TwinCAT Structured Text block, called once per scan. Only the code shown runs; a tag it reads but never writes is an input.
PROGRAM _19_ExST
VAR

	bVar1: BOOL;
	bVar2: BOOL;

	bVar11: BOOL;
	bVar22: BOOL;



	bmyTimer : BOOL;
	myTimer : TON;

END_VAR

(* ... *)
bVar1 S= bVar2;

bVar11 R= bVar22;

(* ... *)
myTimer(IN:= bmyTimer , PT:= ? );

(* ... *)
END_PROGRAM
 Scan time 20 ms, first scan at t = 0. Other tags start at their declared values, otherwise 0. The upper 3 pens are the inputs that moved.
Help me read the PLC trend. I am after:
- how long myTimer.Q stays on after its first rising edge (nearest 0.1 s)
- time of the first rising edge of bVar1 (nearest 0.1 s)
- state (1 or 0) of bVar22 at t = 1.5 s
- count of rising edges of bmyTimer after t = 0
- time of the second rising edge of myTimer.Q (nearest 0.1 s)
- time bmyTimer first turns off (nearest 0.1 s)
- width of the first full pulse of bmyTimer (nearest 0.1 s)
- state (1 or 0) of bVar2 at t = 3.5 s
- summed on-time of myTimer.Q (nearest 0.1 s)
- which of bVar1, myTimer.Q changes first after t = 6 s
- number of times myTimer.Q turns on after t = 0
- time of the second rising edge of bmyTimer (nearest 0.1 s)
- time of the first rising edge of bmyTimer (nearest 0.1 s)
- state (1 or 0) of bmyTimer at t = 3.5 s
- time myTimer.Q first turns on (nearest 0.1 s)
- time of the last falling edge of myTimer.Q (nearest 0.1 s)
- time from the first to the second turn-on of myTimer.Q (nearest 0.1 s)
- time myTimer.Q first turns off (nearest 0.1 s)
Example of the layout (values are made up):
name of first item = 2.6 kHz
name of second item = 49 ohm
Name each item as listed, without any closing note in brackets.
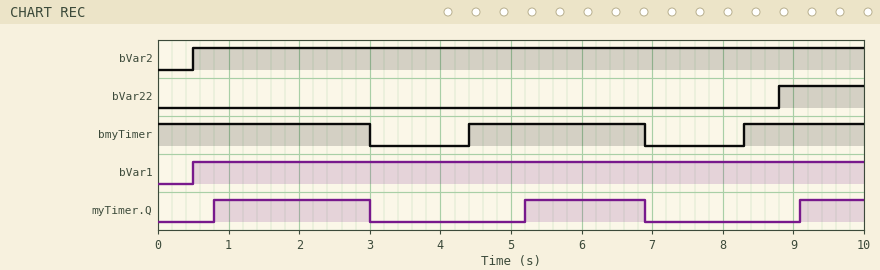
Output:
how long myTimer.Q stays on after its first rising edge = 2.2 s
time of the first rising edge of bVar1 = 0.5 s
state (1 or 0) of bVar22 at t = 1.5 s = 0
count of rising edges of bmyTimer after t = 0 = 2
time of the second rising edge of myTimer.Q = 5.2 s
time bmyTimer first turns off = 3.0 s
width of the first full pulse of bmyTimer = 2.5 s
state (1 or 0) of bVar2 at t = 3.5 s = 1
summed on-time of myTimer.Q = 4.8 s
which of bVar1, myTimer.Q changes first after t = 6 s = myTimer.Q
number of times myTimer.Q turns on after t = 0 = 3
time of the second rising edge of bmyTimer = 8.3 s
time of the first rising edge of bmyTimer = 4.4 s
state (1 or 0) of bmyTimer at t = 3.5 s = 0
time myTimer.Q first turns on = 0.8 s
time of the last falling edge of myTimer.Q = 6.9 s
time from the first to the second turn-on of myTimer.Q = 4.4 s
time myTimer.Q first turns off = 3.0 s
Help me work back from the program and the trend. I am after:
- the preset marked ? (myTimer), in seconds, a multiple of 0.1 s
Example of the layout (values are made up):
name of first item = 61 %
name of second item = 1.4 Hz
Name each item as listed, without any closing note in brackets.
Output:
the preset marked ? (myTimer), in seconds, a multiple of 0.1 s = 0.8 s
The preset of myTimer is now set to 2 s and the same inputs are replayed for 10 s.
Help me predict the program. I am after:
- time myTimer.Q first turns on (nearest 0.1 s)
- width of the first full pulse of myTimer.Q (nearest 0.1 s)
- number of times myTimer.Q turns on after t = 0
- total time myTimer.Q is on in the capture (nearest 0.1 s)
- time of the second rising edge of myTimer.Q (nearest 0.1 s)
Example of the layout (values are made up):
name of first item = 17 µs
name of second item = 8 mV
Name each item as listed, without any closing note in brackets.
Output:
time myTimer.Q first turns on = 2.0 s
width of the first full pulse of myTimer.Q = 1.0 s
number of times myTimer.Q turns on after t = 0 = 2
total time myTimer.Q is on in the capture = 1.5 s
time of the second rising edge of myTimer.Q = 6.4 s
